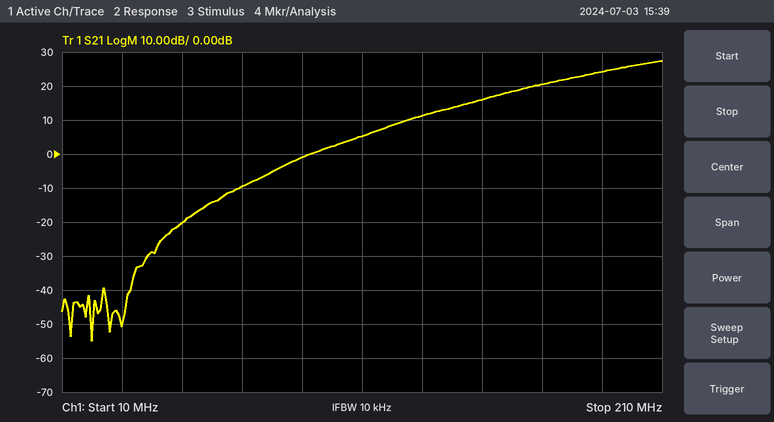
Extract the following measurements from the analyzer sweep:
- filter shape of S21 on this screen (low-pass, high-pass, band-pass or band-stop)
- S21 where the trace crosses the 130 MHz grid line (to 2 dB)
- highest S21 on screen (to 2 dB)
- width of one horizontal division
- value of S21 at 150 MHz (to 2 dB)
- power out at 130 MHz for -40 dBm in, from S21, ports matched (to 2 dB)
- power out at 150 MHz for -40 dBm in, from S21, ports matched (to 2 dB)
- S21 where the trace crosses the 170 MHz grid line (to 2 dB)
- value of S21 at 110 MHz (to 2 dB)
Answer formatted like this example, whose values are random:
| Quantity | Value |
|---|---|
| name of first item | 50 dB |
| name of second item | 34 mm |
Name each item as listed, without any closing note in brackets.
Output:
| Quantity | Value |
|---|---|
| filter shape of S21 on this screen | high-pass |
| S21 where the trace crosses the 130 MHz grid line | 12 dB |
| highest S21 on screen | 28 dB |
| width of one horizontal division | 20 MHz |
| value of S21 at 150 MHz | 16 dB |
| power out at 130 MHz for -40 dBm in, from S21, ports matched | -28 dBm |
| power out at 150 MHz for -40 dBm in, from S21, ports matched | -24 dBm |
| S21 where the trace crosses the 170 MHz grid line | 20 dB |
| value of S21 at 110 MHz | 6 dB |
